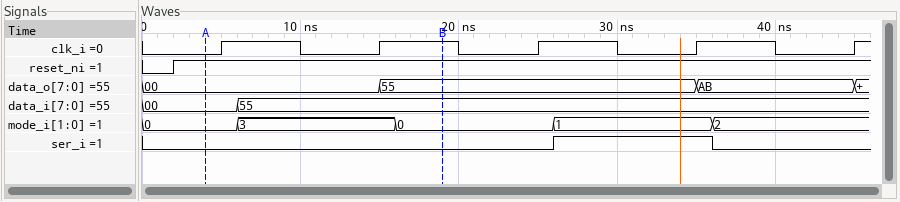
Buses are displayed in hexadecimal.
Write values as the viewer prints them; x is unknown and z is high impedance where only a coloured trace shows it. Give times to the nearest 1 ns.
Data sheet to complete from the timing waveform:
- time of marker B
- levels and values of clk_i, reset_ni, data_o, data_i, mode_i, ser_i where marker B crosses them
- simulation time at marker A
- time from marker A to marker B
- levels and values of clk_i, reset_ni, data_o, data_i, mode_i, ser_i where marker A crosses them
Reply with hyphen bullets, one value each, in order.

- 19 ns
- clk_i=1, reset_ni=1, data_o=55, data_i=55, mode_i=0, ser_i=0
- 4 ns
- 15 ns
- clk_i=0, reset_ni=1, data_o=00, data_i=00, mode_i=0, ser_i=0
